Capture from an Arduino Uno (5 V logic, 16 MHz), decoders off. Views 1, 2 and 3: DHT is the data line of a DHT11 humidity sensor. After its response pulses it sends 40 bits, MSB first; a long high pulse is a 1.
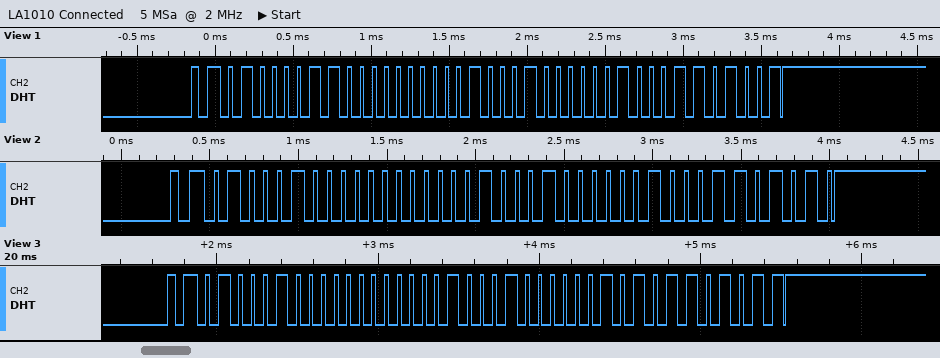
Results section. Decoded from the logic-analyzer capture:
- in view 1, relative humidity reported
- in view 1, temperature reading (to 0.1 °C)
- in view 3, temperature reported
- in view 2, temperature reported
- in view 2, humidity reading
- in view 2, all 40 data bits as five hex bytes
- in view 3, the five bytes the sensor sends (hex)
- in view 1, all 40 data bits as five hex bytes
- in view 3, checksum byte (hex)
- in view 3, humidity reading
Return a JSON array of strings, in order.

["67 %", "34.4 °C", "34.5 °C", "34.4 °C", "68 %", "44 00 22 04 6A", "44 00 22 05 6B", "43 00 22 04 69", "0x6B", "68 %"]
